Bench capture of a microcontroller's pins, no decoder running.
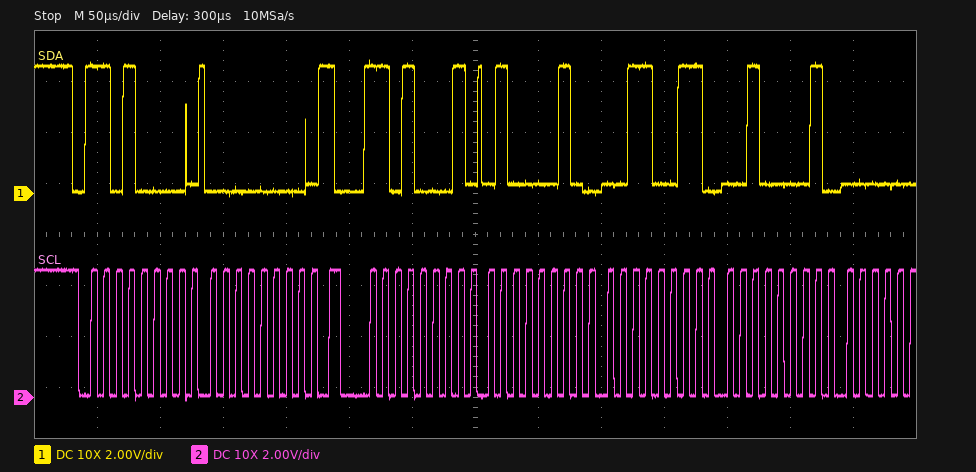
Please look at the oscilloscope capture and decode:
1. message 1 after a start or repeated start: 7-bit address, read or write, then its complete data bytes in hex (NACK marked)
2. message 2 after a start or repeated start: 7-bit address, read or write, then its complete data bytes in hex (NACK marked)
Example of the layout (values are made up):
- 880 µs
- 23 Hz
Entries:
- 0x68 write: 00
- 0x68 read: 42 33 21
